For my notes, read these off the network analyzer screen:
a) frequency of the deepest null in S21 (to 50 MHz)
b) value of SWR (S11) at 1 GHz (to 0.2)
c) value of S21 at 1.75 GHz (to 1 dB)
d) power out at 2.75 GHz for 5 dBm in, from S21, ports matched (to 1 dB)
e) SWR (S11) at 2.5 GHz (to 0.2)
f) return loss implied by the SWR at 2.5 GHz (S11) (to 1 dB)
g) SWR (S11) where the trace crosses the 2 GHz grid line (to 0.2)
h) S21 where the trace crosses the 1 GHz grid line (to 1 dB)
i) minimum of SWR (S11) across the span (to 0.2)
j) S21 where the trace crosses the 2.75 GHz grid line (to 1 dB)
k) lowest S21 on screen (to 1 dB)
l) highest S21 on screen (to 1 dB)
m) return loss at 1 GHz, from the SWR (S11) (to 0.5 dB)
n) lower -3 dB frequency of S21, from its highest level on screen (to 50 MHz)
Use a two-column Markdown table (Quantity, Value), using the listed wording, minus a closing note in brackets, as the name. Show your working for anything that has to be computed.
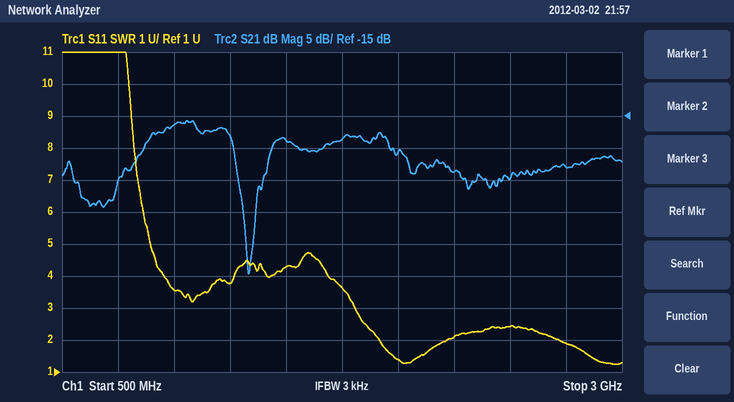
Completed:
| Quantity | Value |
|---|---|
| frequency of the deepest null in S21 | 1.35 GHz |
| value of SWR (S11) at 1 GHz | 3.6 |
| value of S21 at 1.75 GHz | -19 dB |
| power out at 2.75 GHz for 5 dBm in, from S21, ports matched | 5 dBm + (-23 dB) = -18 dBm |
| SWR (S11) at 2.5 GHz | 2.4 |
| return loss implied by the SWR at 2.5 GHz (S11) | −20 log10((2.4 − 1)/(2.4 + 1)) ≈ 8 dB |
| SWR (S11) where the trace crosses the 2 GHz grid line | 1.4 |
| S21 where the trace crosses the 1 GHz grid line | -16 dB |
| minimum of SWR (S11) across the span | 1.2 |
| S21 where the trace crosses the 2.75 GHz grid line | -23 dB |
| lowest S21 on screen | -40 dB |
| highest S21 on screen | -16 dB |
| return loss at 1 GHz, from the SWR (S11) | −20 log10((3.6 − 1)/(3.6 + 1)) ≈ 5.0 dB |
| lower -3 dB frequency of S21, from its highest level on screen | 900 MHz |
